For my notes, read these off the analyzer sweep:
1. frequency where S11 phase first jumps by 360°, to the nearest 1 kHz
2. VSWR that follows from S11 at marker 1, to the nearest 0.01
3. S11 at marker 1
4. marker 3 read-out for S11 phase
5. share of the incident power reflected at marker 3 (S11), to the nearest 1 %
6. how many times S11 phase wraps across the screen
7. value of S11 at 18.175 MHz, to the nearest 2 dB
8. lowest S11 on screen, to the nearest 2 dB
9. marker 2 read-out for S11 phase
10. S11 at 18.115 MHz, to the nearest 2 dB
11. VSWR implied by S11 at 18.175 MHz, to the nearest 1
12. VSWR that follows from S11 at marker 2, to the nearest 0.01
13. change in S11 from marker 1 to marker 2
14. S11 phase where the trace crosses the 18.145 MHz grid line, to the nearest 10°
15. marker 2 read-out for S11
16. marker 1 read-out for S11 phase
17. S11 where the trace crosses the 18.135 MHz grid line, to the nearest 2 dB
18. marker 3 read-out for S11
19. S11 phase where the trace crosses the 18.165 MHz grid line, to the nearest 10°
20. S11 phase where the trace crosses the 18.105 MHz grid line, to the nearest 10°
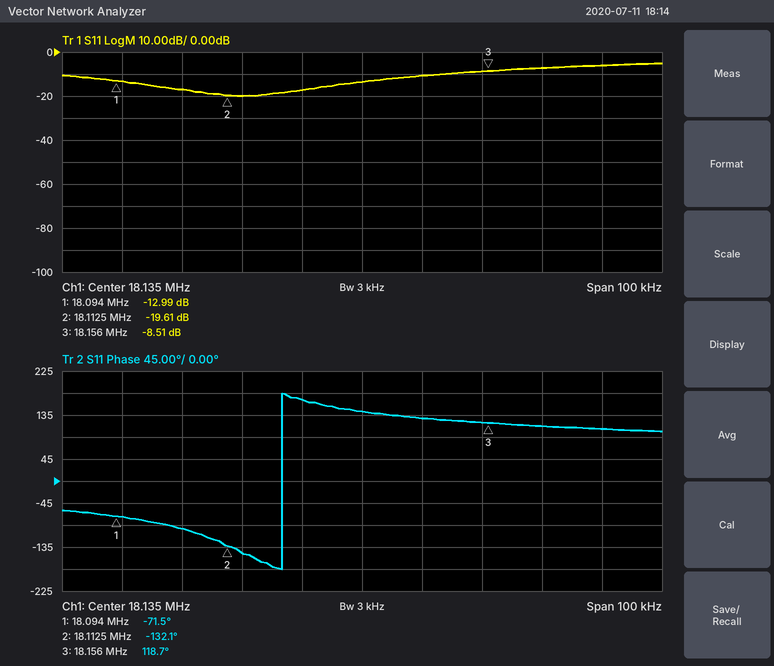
18.122 MHz
1.58
-12.99 dB
118.7°
14 %
1
-6 dB
-20 dB
-132.1°
-20 dB
3
1.23
-6.62 dB
130°
-19.61 dB
-71.5°
-14 dB
-8.51 dB
110°
-100°
